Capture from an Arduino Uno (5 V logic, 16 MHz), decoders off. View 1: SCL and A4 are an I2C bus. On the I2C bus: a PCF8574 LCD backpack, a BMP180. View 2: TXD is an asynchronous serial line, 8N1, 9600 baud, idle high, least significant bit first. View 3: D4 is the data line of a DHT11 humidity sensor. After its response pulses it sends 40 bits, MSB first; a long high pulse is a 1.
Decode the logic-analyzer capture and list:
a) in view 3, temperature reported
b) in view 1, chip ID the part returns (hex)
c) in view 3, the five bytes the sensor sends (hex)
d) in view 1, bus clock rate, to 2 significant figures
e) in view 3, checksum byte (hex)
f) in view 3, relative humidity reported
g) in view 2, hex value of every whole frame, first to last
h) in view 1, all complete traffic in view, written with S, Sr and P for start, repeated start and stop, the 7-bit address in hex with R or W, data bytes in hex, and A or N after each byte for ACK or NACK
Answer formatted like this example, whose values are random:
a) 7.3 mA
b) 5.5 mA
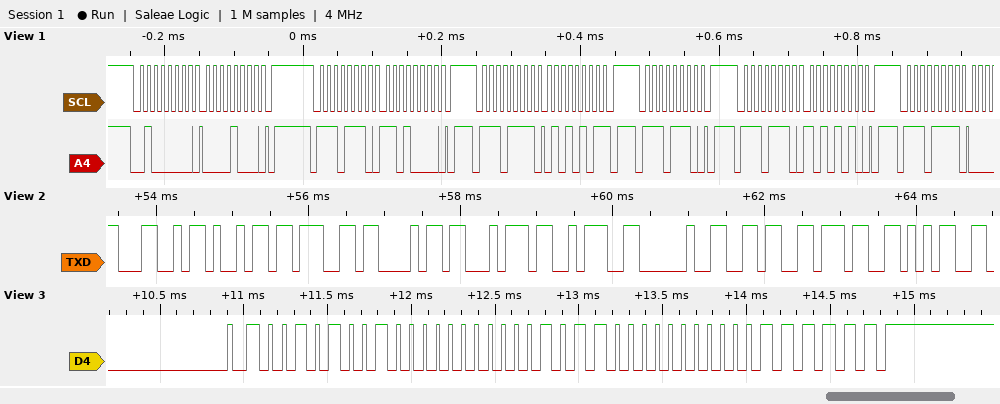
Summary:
a) 22.0 °C
b) 0x55
c) 29 00 16 00 3F
d) 100 kHz
e) 0x3F
f) 41 %
g) 4C 69 67 68 74 3A 20 36 37 35
h) S 20W A 08 A P S 77W A D0 A P S 77R A 55 N P S 77W A P S 77W A AA A P S 77R A
